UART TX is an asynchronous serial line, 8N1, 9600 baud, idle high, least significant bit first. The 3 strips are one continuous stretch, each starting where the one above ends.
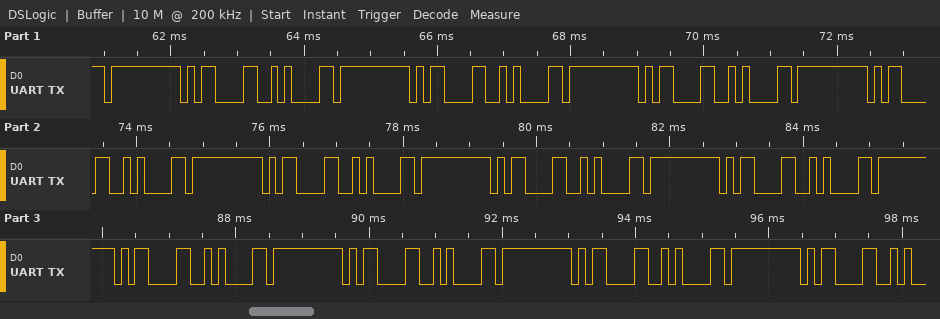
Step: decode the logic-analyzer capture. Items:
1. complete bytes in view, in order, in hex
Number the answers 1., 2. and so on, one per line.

1. FF 0D 0A FF 0D 0A FF 0D 0A FF 0D 0A FF 0D 0A FF 0D 0A FF 0D 0A FF 0D 0A FF 0D 0A FF 0D 0A FF 0D
